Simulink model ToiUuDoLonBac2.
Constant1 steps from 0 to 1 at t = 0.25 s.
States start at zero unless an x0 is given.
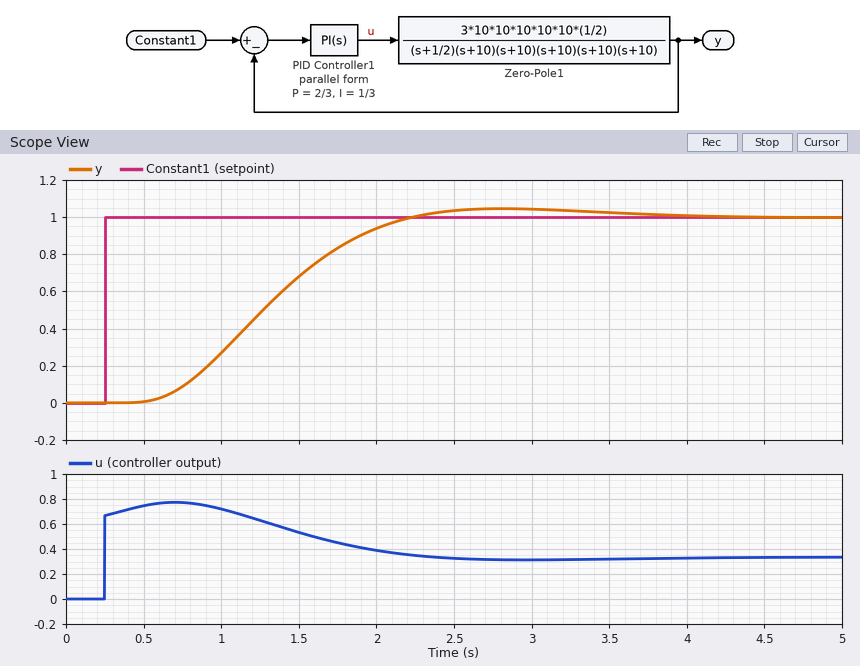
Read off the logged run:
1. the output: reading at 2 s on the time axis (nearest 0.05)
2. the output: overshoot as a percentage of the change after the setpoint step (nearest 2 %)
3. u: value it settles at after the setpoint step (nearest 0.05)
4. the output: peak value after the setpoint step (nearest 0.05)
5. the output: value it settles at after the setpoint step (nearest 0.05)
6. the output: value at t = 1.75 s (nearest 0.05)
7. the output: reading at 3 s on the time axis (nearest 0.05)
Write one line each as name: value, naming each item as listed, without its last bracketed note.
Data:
the output: reading at 2 s on the time axis: 0.95
the output: overshoot as a percentage of the change after the setpoint step: 4 %
u: value it settles at after the setpoint step: 0.35
the output: peak value after the setpoint step: 1.05
the output: value it settles at after the setpoint step: 1.00
the output: value at t = 1.75 s: 0.85
the output: reading at 3 s on the time axis: 1.05
